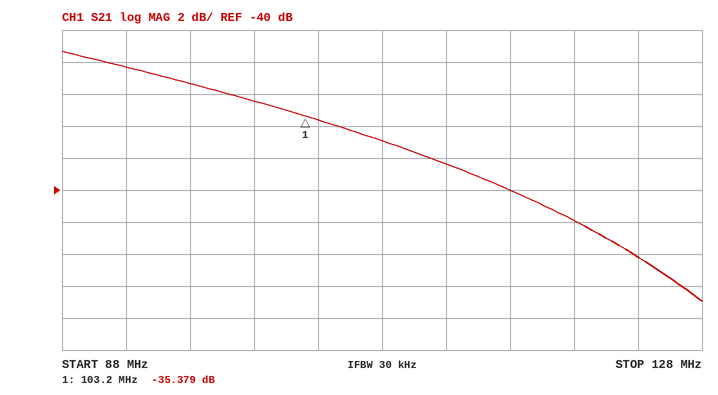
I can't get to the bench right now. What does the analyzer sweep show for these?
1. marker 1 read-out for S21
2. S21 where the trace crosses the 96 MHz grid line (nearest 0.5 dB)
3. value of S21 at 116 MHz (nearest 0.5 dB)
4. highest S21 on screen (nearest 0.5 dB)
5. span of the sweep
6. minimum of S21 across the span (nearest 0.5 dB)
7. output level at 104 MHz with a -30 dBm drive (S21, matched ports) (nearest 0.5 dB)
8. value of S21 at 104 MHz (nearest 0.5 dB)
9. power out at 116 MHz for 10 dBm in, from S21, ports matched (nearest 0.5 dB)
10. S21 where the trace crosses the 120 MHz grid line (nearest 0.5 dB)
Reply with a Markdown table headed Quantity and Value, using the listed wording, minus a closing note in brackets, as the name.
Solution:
| Quantity | Value |
|---|---|
| marker 1 read-out for S21 | -35.379 dB |
| S21 where the trace crosses the 96 MHz grid line | -33.5 dB |
| value of S21 at 116 MHz | -40.0 dB |
| highest S21 on screen | -31.5 dB |
| span of the sweep | 40 MHz |
| minimum of S21 across the span | -47.0 dB |
| output level at 104 MHz with a -30 dBm drive (S21, matched ports) | -65.5 dBm |
| value of S21 at 104 MHz | -35.5 dB |
| power out at 116 MHz for 10 dBm in, from S21, ports matched | -30.0 dBm |
| S21 where the trace crosses the 120 MHz grid line | -42.0 dB |
